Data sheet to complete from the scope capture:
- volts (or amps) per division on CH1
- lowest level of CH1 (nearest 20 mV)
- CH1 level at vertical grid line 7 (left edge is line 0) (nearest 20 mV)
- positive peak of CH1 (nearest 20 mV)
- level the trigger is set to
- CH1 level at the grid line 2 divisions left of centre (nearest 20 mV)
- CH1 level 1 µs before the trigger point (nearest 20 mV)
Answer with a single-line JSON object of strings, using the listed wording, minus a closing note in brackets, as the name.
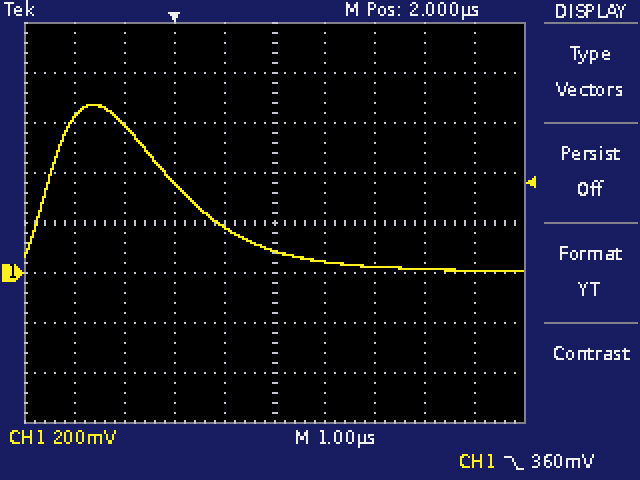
{"volts (or amps) per division on CH1": "200 mV", "lowest level of CH1": "0 mV", "CH1 level at vertical grid line 7 (left edge is line 0)": "20 mV", "positive peak of CH1": "680 mV", "level the trigger is set to": "360 mV", "CH1 level at the grid line 2 divisions left of centre": "360 mV", "CH1 level 1 µs before the trigger point": "600 mV"}
